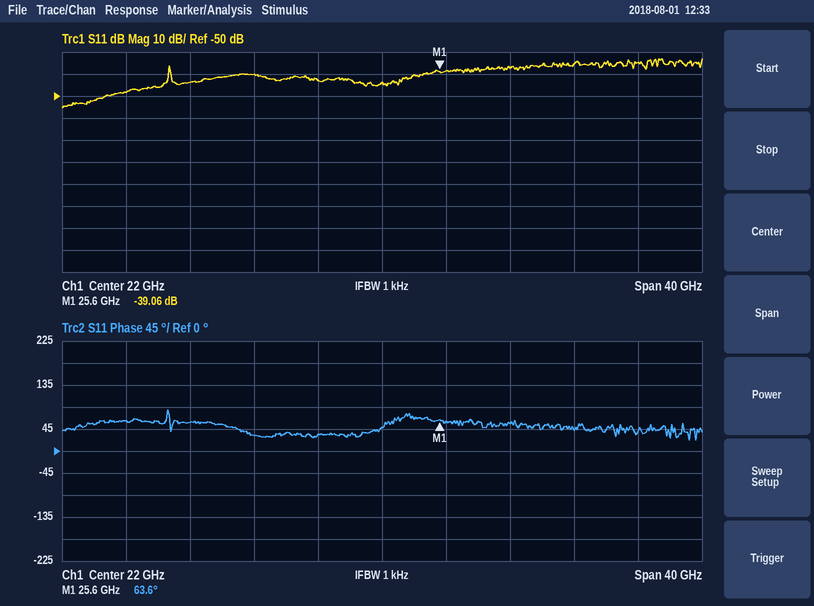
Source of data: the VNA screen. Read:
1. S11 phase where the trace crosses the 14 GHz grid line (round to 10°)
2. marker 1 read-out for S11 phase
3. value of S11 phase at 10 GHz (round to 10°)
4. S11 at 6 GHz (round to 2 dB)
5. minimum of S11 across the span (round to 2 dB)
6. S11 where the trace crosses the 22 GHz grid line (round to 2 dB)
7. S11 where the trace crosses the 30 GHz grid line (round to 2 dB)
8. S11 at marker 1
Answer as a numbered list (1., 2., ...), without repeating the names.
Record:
1. 30°
2. 63.6°
3. 60°
4. -48 dB
5. -56 dB
6. -44 dB
7. -38 dB
8. -39.06 dB
